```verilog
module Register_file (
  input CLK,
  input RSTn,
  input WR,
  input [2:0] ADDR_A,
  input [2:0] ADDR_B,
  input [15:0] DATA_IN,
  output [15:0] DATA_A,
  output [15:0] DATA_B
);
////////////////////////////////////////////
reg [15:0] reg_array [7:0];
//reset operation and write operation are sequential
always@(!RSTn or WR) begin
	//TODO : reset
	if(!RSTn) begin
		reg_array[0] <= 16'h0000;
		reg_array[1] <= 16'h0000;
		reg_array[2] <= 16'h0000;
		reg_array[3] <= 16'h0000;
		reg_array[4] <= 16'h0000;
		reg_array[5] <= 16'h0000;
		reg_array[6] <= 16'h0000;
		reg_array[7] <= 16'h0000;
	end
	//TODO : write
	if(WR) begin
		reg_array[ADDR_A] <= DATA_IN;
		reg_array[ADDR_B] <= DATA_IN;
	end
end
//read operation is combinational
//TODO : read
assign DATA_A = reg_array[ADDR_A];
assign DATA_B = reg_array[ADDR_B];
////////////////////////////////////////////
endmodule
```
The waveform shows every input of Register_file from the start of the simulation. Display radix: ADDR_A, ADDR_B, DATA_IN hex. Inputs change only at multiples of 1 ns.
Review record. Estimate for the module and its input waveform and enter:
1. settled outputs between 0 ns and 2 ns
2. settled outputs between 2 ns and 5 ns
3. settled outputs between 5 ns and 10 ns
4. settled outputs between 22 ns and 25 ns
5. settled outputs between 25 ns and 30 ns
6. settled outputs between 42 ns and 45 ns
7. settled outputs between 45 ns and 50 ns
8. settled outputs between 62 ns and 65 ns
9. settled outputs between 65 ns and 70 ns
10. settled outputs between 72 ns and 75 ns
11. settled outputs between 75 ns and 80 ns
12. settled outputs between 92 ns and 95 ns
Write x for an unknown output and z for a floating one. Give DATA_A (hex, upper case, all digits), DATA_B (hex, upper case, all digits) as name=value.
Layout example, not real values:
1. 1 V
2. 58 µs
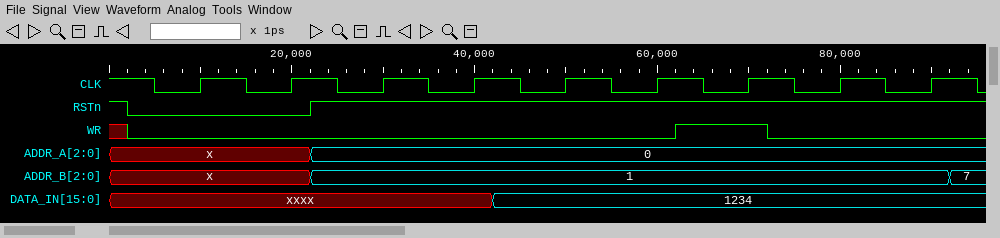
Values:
1. DATA_A=x, DATA_B=x
2. DATA_A=x, DATA_B=x
3. DATA_A=x, DATA_B=x
4. DATA_A=0000, DATA_B=0000
5. DATA_A=0000, DATA_B=0000
6. DATA_A=0000, DATA_B=0000
7. DATA_A=0000, DATA_B=0000
8. DATA_A=1234, DATA_B=1234
9. DATA_A=1234, DATA_B=1234
10. DATA_A=1234, DATA_B=1234
11. DATA_A=1234, DATA_B=1234
12. DATA_A=1234, DATA_B=0000
